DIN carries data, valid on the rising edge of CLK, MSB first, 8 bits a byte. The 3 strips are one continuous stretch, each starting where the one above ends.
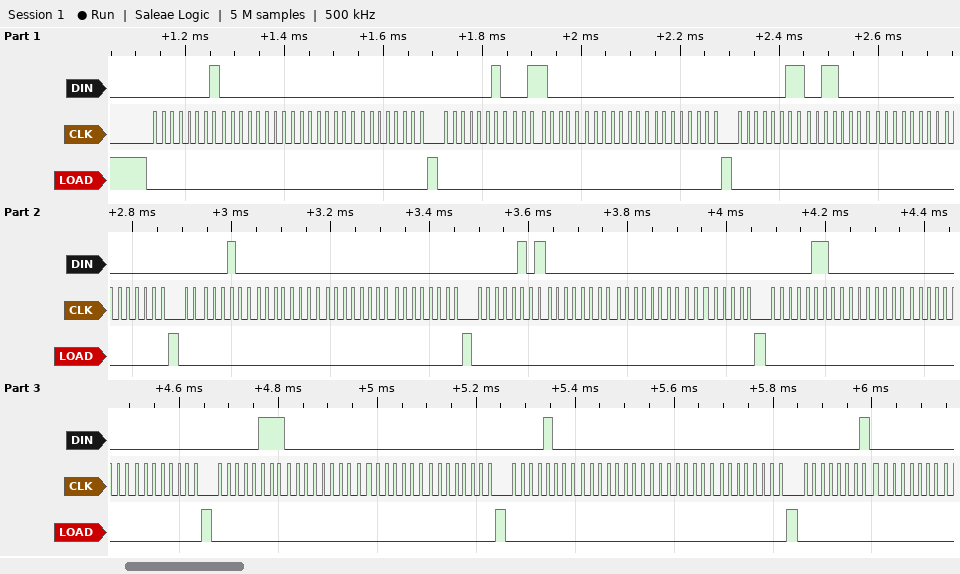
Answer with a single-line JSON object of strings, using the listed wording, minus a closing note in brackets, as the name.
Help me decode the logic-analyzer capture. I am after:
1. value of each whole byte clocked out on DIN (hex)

{"value of each whole byte clocked out on DIN": "0x01 0x00 0x00 0x00 0x02 0x30 0x00 0x00 0x03 0x30 0x00 0x00 0x04 0x00 0x00 0x00 0x05 0x00 0x00 0x00 0x06 0x00 0x00 0x00 0x07 0x00 0x00 0x00 0x08 0x00 0x00 0x00 0x01 0x00"}
